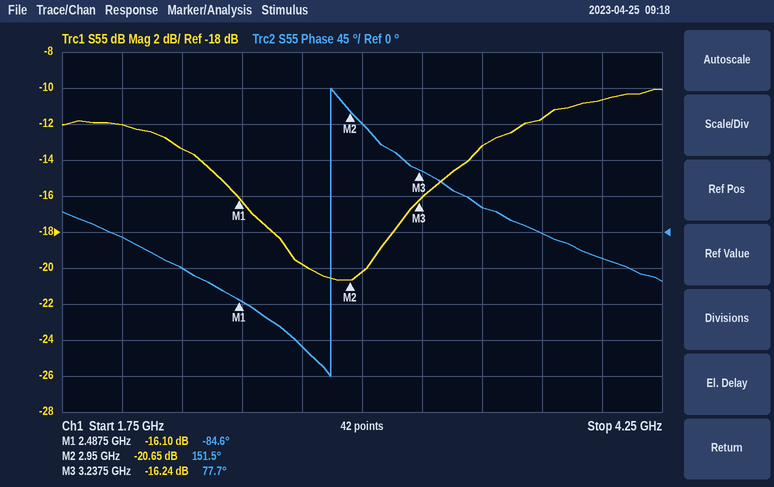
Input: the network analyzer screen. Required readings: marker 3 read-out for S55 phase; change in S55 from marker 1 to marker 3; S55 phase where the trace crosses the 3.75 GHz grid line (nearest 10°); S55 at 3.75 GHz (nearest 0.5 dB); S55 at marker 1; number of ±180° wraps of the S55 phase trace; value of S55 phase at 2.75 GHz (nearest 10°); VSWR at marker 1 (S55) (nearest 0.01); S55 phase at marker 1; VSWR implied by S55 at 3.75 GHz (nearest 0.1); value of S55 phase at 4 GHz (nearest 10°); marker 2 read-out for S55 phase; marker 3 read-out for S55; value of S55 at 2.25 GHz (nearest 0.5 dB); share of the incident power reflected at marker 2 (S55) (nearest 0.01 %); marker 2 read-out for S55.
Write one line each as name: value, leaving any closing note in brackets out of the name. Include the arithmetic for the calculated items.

marker 3 read-out for S55 phase: 77.7°
change in S55 from marker 1 to marker 3: -16.24 − (-16.1) = -0.14 dB
S55 phase where the trace crosses the 3.75 GHz grid line: 0°
S55 at 3.75 GHz: -11.5 dB
S55 at marker 1: -16.10 dB
number of ±180° wraps of the S55 phase trace: 1
value of S55 phase at 2.75 GHz: -140°
VSWR at marker 1 (S55): (1 + 0.1567)/(1 − 0.1567) ≈ 1.37
S55 phase at marker 1: -84.6°
VSWR implied by S55 at 3.75 GHz: |Γ| = 10^(-11.5/20) = 0.2661; VSWR = (1 + 0.2661)/(1 − 0.2661) ≈ 1.7
value of S55 phase at 4 GHz: -30°
marker 2 read-out for S55 phase: 151.5°
marker 3 read-out for S55: -16.24 dB
value of S55 at 2.25 GHz: -13.5 dB
share of the incident power reflected at marker 2 (S55): 10^(-20.65/10) ≈ 0.86 %
marker 2 read-out for S55: -20.65 dB
